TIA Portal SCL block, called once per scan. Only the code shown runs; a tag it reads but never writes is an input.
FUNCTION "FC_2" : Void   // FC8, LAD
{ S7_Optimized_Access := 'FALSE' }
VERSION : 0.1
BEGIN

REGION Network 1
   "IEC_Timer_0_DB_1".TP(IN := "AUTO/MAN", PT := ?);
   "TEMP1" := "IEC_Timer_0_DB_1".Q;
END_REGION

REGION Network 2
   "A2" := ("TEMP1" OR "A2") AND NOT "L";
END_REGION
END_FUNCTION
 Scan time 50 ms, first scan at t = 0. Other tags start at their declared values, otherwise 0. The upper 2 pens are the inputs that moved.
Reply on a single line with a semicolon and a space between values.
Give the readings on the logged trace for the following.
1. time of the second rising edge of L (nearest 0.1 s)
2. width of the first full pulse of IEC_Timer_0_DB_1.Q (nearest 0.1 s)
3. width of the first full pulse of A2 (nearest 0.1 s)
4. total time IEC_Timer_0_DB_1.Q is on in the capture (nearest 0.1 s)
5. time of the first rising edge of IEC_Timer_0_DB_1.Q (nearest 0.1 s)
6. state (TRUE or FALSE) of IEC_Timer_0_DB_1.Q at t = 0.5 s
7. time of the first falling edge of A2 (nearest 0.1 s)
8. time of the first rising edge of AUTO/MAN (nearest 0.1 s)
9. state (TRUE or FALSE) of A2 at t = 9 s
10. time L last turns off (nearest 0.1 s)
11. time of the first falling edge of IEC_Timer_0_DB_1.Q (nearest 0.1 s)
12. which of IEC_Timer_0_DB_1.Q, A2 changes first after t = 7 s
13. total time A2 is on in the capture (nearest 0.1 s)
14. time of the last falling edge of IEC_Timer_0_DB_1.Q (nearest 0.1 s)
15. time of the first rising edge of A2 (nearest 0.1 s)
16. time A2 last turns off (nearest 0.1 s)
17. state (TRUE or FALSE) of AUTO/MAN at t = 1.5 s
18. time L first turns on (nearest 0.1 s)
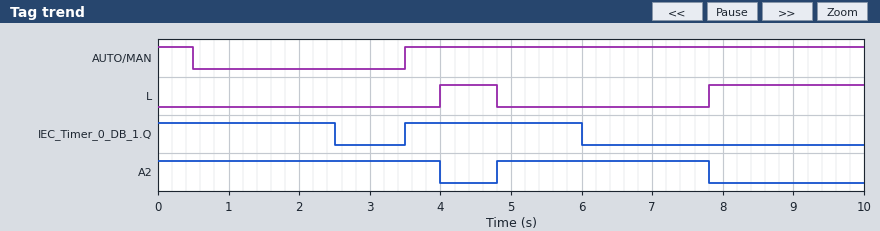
7.8 s; 2.5 s; 3.0 s; 5.0 s; 3.5 s; TRUE; 4.0 s; 3.5 s; FALSE; 4.8 s; 2.5 s; A2; 7.0 s; 6.0 s; 4.8 s; 7.8 s; FALSE; 4.0 s
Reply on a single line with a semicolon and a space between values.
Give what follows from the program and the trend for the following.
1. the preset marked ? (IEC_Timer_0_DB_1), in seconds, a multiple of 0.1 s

2.5 s
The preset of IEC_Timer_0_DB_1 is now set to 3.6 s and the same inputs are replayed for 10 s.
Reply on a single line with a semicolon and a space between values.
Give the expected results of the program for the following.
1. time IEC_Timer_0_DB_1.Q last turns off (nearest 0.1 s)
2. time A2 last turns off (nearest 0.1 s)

3.6 s; 4.0 s
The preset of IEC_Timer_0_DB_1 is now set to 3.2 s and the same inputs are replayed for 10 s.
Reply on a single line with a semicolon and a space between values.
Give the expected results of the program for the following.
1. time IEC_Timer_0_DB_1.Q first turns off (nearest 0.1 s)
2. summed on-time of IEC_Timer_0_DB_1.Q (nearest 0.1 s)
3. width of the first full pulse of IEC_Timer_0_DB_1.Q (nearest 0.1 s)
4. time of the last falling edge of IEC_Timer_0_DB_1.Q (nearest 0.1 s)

3.2 s; 6.4 s; 3.2 s; 6.7 s
